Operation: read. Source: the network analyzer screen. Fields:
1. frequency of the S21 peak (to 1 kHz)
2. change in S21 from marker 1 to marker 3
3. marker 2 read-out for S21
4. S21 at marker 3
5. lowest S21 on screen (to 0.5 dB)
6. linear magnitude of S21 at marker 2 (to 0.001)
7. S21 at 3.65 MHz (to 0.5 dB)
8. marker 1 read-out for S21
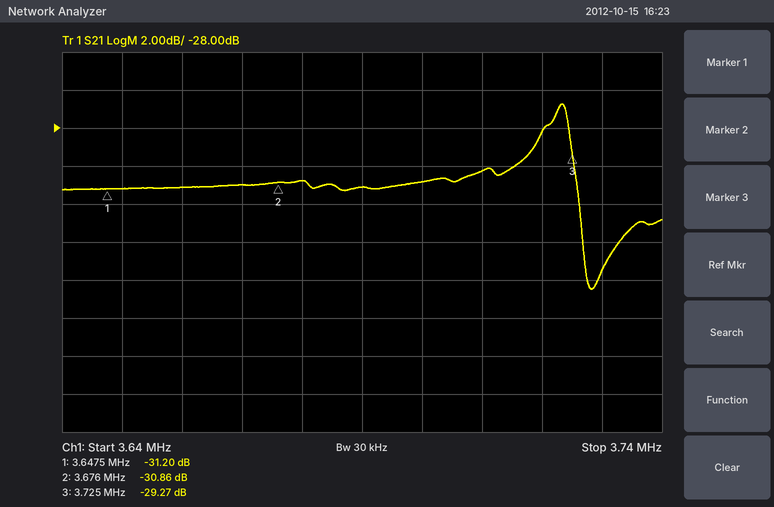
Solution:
3.723 MHz
1.93 dB
-30.86 dB
-29.27 dB
-36.5 dB
0.029
-31.0 dB
-31.20 dB
